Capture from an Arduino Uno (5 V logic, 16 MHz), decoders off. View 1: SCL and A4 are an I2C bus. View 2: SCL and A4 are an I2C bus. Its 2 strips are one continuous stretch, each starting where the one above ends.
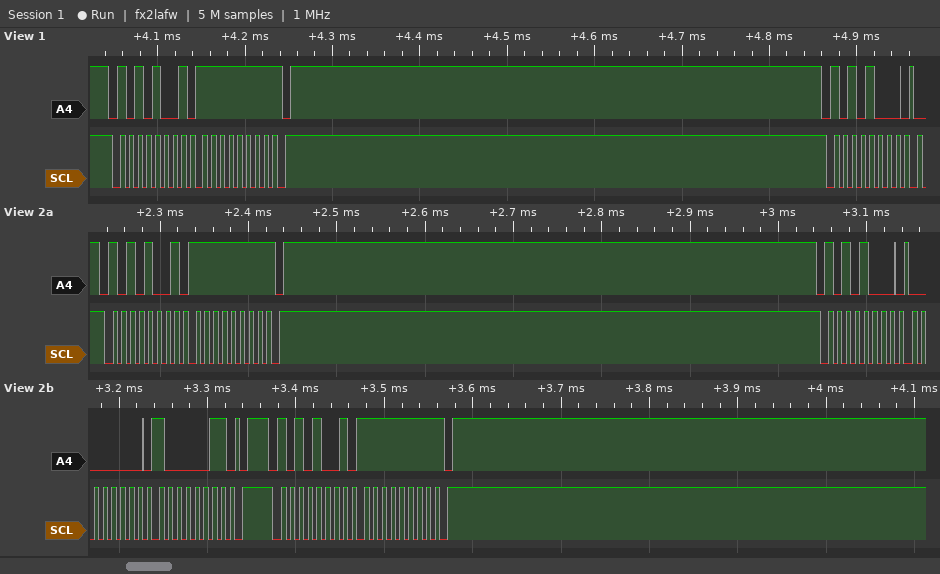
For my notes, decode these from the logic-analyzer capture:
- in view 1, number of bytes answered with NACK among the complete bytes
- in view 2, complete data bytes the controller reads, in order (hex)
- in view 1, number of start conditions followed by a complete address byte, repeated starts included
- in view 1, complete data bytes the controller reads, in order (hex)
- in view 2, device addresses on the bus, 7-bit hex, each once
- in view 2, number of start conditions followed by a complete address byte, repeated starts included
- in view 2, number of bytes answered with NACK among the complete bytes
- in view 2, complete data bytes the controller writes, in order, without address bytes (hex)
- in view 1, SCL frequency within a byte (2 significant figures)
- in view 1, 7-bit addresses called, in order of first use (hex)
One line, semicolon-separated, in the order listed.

1; FF FF; 2; FF; 0x54; 3; 2; 00 83; 100 kHz; 0x54
